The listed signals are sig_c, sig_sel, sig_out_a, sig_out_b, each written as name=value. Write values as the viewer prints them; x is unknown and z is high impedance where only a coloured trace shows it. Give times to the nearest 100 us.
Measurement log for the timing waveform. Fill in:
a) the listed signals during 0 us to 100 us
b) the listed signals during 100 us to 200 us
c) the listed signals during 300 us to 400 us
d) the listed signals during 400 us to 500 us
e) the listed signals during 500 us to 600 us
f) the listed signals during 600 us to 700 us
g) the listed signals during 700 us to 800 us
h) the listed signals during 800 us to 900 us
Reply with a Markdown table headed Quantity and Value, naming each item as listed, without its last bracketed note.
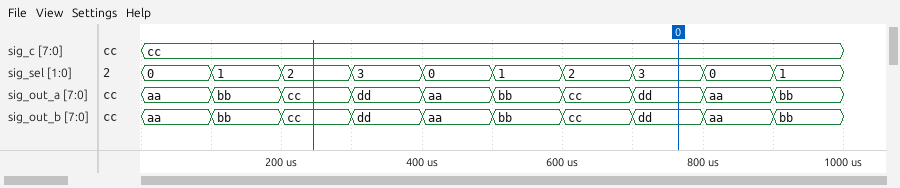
| Quantity | Value |
|---|---|
| the listed signals during 0 us to 100 us | sig_c=cc, sig_sel=0, sig_out_a=aa, sig_out_b=aa |
| the listed signals during 100 us to 200 us | sig_c=cc, sig_sel=1, sig_out_a=bb, sig_out_b=bb |
| the listed signals during 300 us to 400 us | sig_c=cc, sig_sel=3, sig_out_a=dd, sig_out_b=dd |
| the listed signals during 400 us to 500 us | sig_c=cc, sig_sel=0, sig_out_a=aa, sig_out_b=aa |
| the listed signals during 500 us to 600 us | sig_c=cc, sig_sel=1, sig_out_a=bb, sig_out_b=bb |
| the listed signals during 600 us to 700 us | sig_c=cc, sig_sel=2, sig_out_a=cc, sig_out_b=cc |
| the listed signals during 700 us to 800 us | sig_c=cc, sig_sel=3, sig_out_a=dd, sig_out_b=dd |
| the listed signals during 800 us to 900 us | sig_c=cc, sig_sel=0, sig_out_a=aa, sig_out_b=aa |
